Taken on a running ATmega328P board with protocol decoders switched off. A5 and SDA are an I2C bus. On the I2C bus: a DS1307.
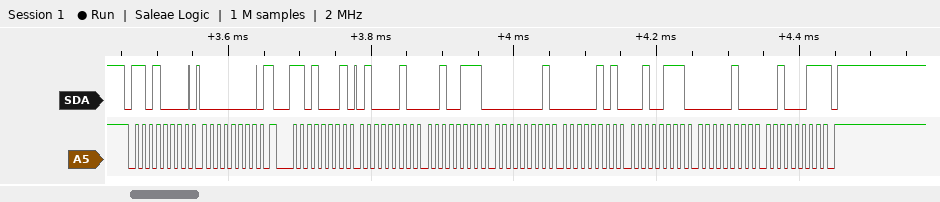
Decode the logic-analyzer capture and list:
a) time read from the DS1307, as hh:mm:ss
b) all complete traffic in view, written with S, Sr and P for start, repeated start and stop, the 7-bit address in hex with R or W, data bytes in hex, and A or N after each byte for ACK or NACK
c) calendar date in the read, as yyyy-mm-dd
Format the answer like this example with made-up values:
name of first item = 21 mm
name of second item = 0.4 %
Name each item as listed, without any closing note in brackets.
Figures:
time read from the DS1307, as hh:mm:ss = 01:27:42
all complete traffic in view, written with S, Sr and P for start, repeated start and stop, the 7-bit address in hex with R or W, data bytes in hex, and A or N after each byte for ACK or NACK = S 68W A 00 A Sr 68R A 42 A 27 A 01 A 05 A 27 A 04 A 23 N P
calendar date in the read, as yyyy-mm-dd = 2023-04-27
